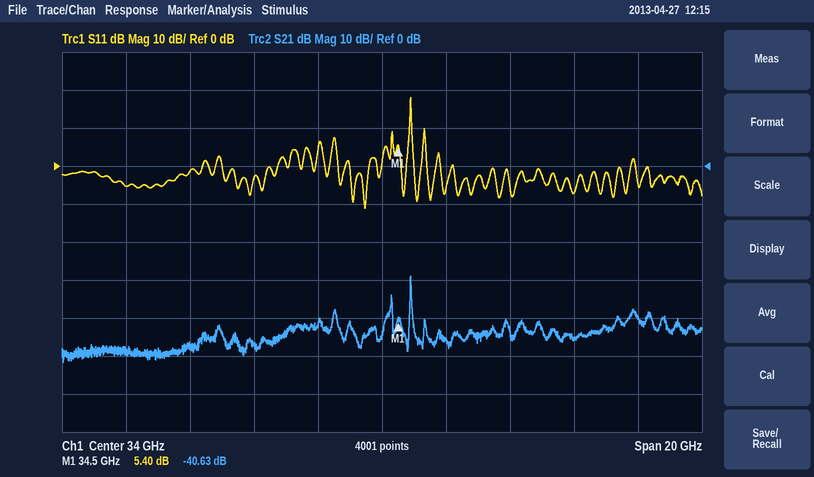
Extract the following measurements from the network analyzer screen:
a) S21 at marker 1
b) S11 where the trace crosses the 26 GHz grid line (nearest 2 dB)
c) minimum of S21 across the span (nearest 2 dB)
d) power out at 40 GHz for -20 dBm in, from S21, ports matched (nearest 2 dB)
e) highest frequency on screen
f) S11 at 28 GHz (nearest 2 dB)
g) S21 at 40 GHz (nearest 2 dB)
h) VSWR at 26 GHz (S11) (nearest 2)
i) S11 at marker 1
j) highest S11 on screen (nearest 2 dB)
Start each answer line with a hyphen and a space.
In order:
- -40.63 dB
- -6 dB
- -52 dB
- -66 dBm
- 44 GHz
- -2 dB
- -46 dB
- 4
- 5.40 dB
- 18 dB
